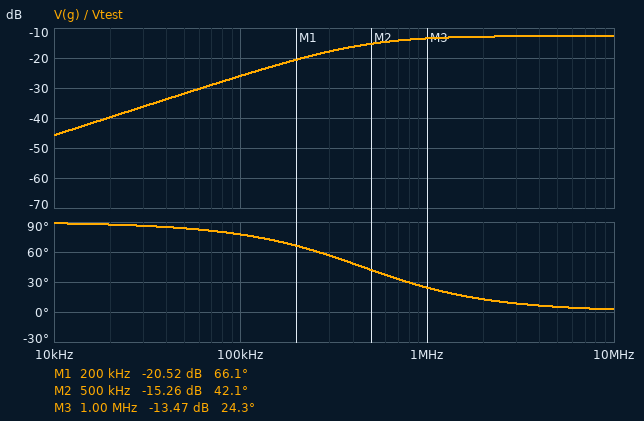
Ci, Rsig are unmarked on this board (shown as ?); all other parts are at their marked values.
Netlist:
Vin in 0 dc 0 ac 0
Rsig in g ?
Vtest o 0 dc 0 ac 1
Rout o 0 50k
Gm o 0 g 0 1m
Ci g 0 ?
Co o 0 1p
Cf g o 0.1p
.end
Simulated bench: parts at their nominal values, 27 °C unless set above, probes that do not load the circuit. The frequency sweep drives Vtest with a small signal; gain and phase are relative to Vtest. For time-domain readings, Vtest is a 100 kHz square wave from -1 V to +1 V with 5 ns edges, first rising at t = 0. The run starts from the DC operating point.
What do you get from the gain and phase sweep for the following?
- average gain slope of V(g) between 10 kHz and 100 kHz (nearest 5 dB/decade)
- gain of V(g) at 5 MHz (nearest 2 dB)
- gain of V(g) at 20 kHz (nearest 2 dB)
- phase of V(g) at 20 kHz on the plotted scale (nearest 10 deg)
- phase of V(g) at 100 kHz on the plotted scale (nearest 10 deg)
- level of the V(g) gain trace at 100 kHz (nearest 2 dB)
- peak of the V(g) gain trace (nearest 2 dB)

20 dB/decade
-12 dB
-40 dB
90 deg
80 deg
-26 dB
-12 dB
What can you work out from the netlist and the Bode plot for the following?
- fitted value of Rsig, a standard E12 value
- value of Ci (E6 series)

820 kΩ
330 fF
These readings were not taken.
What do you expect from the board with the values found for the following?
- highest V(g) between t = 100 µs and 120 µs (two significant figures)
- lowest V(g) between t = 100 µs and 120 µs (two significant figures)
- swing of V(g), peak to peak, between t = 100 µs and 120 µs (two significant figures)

460 mV
-460 mV
920 mV
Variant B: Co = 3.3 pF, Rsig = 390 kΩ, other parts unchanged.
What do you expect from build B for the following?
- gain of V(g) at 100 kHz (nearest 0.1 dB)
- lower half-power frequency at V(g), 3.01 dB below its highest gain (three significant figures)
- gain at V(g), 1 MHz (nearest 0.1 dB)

-32.3 dB
949 kHz
-15.5 dB
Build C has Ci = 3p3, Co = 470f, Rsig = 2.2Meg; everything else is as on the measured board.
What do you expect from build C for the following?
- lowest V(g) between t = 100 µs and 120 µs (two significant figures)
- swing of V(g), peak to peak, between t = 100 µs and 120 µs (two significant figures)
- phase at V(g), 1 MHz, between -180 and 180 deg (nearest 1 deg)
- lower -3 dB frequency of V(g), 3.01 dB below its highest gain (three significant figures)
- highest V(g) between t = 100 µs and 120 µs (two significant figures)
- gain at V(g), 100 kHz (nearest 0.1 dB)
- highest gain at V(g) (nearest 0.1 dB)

-39 mV
78 mV
1 deg
21.3 kHz
39 mV
-30.8 dB
-30.6 dB
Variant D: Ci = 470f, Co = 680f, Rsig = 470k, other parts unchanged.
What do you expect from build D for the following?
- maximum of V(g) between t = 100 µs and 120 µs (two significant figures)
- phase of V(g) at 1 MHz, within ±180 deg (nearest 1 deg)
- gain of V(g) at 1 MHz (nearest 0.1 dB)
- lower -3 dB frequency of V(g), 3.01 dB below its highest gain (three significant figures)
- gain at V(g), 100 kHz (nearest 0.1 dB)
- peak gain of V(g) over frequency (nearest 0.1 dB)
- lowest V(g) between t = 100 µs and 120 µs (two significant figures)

350 mV
31 deg
-16.4 dB
594 kHz
-30.7 dB
-15.1 dB
-350 mV
